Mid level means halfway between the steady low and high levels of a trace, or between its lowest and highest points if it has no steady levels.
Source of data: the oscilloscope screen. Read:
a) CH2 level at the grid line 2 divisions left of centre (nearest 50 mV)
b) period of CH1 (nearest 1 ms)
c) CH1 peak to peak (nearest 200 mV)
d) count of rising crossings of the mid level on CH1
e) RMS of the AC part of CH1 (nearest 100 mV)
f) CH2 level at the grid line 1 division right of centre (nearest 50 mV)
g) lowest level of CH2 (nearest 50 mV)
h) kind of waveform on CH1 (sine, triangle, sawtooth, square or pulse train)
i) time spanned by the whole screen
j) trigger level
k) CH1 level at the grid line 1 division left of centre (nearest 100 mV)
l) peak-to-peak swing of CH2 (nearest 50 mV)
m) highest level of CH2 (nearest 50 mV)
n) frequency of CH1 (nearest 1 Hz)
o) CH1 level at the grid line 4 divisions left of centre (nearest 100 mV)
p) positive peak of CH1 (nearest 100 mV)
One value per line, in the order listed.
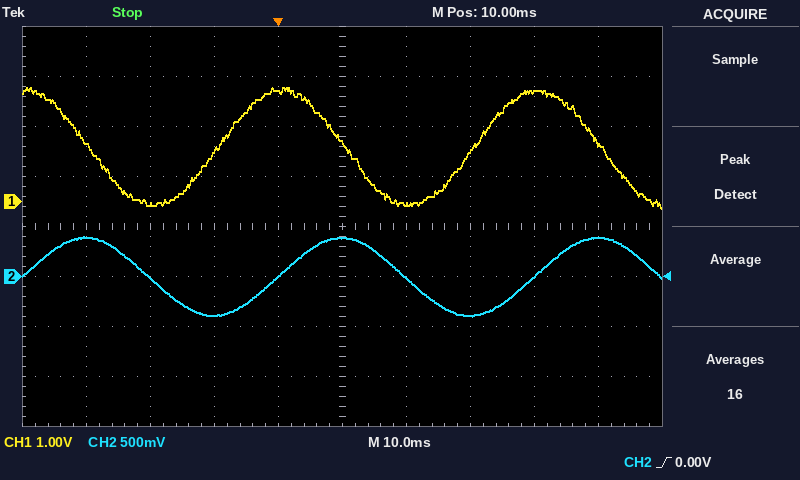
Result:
-400 mV
40 ms
2.4 V
2
800 mV
0 mV
-400 mV
sine
100 ms
0.00 V
2.2 V
800 mV
400 mV
25 Hz
1.2 V
2.3 V
